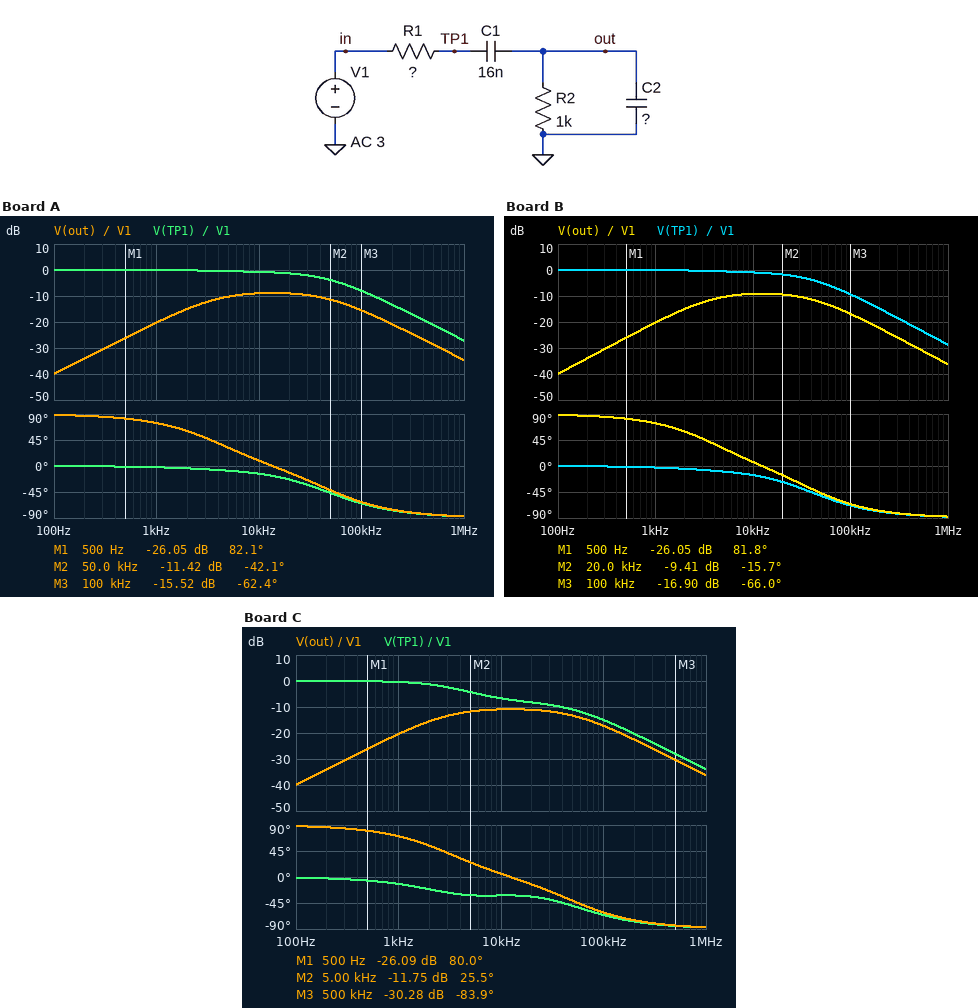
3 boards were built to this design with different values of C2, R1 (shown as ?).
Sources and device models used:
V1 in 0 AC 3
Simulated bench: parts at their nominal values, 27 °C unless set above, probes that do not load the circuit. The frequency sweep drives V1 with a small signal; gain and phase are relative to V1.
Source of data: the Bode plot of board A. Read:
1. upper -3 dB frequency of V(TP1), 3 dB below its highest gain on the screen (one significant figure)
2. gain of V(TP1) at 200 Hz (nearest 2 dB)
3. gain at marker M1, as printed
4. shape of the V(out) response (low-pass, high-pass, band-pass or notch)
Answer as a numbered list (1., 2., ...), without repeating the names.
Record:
1. 40 kHz
2. 0 dB
3. -26.05 dB
4. band-pass
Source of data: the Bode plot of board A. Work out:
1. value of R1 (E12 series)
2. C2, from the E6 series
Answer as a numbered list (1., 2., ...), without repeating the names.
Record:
1. 390 Ω
2. 22 nF
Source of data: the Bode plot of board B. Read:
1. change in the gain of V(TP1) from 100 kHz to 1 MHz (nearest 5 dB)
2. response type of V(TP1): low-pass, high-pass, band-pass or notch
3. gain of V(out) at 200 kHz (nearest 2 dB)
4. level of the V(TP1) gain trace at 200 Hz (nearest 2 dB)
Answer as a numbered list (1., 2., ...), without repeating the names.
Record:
1. -20 dB
2. low-pass
3. -22 dB
4. 0 dB
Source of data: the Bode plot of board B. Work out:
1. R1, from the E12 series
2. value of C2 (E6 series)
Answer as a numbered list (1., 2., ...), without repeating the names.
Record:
1. 470 Ω
2. 22 nF
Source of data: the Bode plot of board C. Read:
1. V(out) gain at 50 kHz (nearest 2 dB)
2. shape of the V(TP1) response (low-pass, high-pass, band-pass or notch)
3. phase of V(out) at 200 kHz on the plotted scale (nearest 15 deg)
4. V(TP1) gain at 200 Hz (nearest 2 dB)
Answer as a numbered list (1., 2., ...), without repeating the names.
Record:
1. -14 dB
2. low-pass
3. -75 deg
4. 0 dB
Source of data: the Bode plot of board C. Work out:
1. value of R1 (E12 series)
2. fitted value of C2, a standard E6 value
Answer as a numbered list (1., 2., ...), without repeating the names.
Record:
1. 2.2 kΩ
2. 4.7 nF
